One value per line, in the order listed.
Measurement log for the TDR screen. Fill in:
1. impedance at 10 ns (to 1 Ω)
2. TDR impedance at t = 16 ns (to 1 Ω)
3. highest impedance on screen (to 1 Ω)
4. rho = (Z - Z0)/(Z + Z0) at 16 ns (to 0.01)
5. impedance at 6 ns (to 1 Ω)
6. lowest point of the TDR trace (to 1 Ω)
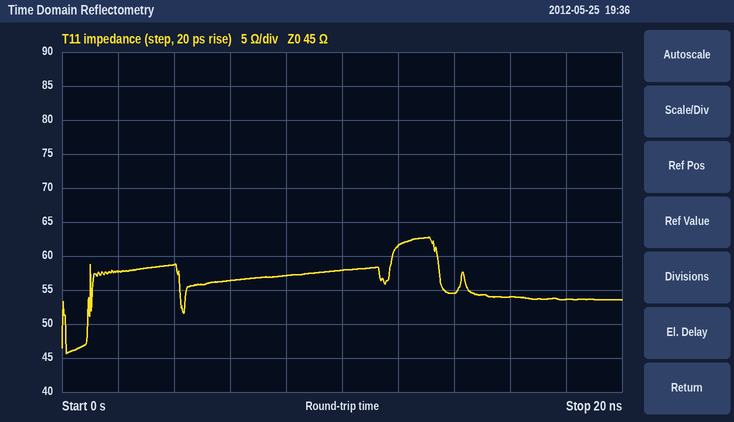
58 Ω
54 Ω
63 Ω
+0.09
56 Ω
46 Ω
